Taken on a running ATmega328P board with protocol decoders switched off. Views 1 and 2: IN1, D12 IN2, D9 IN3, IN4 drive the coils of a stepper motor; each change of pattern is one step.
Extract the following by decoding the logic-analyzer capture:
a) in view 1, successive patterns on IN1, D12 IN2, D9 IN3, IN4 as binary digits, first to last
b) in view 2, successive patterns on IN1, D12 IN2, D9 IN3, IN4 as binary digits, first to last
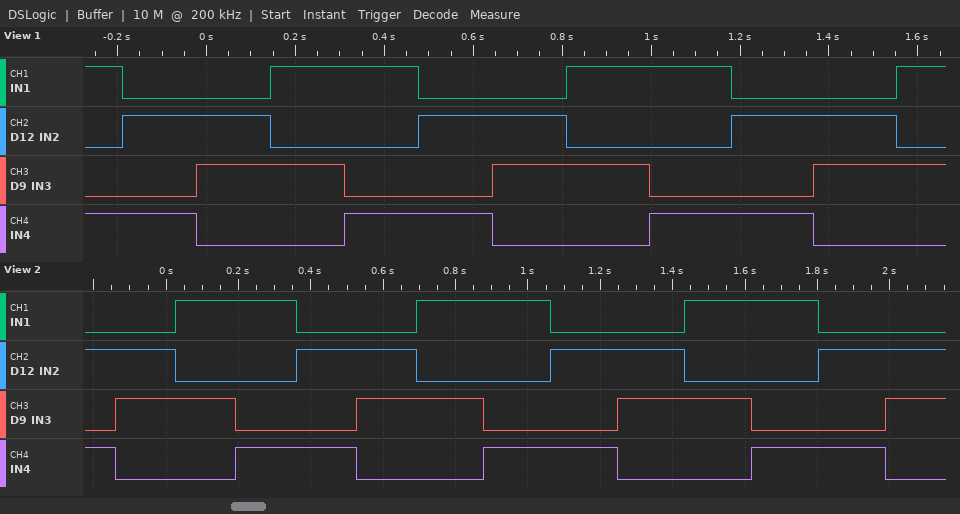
1001 0101 0110 1010 1001 0101 0110 1010 1001 0101 0110 1010
0101 0110 1010 1001 0101 0110 1010 1001 0101 0110 1010 1001 0101 0110
